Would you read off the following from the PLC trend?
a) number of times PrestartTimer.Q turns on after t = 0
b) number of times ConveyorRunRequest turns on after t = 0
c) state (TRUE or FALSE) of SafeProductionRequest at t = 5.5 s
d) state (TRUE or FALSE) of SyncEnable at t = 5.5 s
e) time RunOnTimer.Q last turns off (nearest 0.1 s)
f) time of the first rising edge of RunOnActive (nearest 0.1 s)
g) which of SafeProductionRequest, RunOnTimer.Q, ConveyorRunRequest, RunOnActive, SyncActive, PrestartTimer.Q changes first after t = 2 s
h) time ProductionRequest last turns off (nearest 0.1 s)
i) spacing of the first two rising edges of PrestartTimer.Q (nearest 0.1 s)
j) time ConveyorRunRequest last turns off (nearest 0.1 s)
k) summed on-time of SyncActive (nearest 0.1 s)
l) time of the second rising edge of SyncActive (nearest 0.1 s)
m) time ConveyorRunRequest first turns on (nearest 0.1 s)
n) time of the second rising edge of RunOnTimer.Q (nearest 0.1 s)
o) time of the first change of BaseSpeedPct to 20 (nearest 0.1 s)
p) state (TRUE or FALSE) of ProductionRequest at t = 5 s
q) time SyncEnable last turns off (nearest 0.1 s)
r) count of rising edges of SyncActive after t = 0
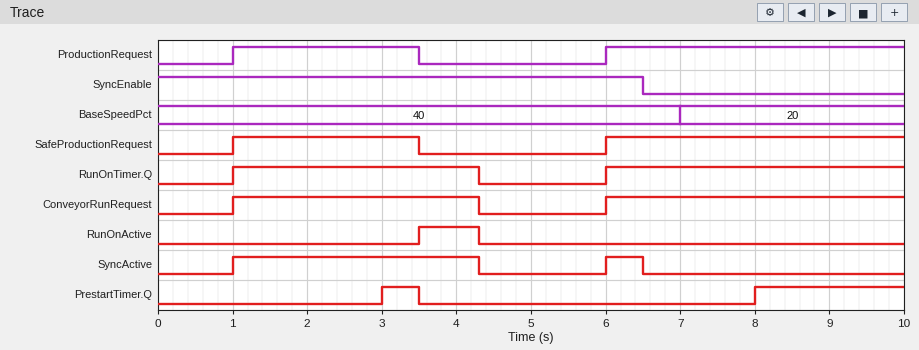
2
2
FALSE
TRUE
4.3 s
3.5 s
PrestartTimer.Q
3.5 s
5.0 s
4.3 s
3.8 s
6.0 s
1.0 s
6.0 s
7.0 s
FALSE
6.5 s
2
